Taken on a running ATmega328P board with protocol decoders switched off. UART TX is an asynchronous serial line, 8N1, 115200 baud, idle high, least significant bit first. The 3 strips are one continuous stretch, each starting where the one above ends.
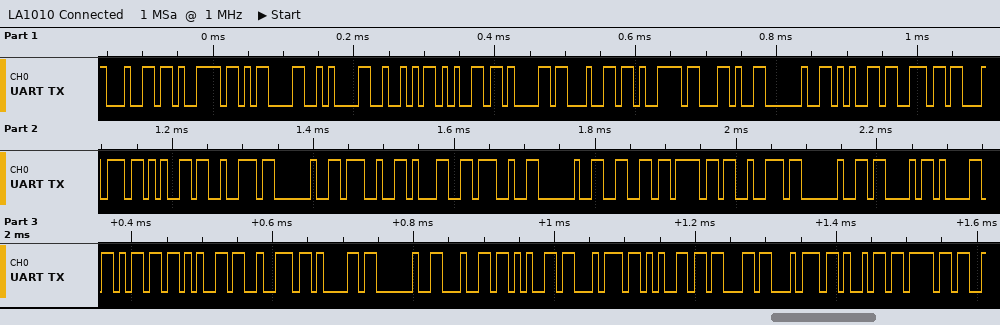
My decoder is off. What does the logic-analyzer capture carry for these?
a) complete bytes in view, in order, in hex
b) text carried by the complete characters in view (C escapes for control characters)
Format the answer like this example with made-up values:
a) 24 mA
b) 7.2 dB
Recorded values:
a) 64 79 0D 0A 52 65 61 64 79 2C 20 65 6E 74 65 72 20 27 31 27 20 66 6F 72 20 43 61 6D 65 72 61 20 64 65 74 65 63 74 69 6F
b) "dy\r\nReady, enter '1' for Camera detectio"
